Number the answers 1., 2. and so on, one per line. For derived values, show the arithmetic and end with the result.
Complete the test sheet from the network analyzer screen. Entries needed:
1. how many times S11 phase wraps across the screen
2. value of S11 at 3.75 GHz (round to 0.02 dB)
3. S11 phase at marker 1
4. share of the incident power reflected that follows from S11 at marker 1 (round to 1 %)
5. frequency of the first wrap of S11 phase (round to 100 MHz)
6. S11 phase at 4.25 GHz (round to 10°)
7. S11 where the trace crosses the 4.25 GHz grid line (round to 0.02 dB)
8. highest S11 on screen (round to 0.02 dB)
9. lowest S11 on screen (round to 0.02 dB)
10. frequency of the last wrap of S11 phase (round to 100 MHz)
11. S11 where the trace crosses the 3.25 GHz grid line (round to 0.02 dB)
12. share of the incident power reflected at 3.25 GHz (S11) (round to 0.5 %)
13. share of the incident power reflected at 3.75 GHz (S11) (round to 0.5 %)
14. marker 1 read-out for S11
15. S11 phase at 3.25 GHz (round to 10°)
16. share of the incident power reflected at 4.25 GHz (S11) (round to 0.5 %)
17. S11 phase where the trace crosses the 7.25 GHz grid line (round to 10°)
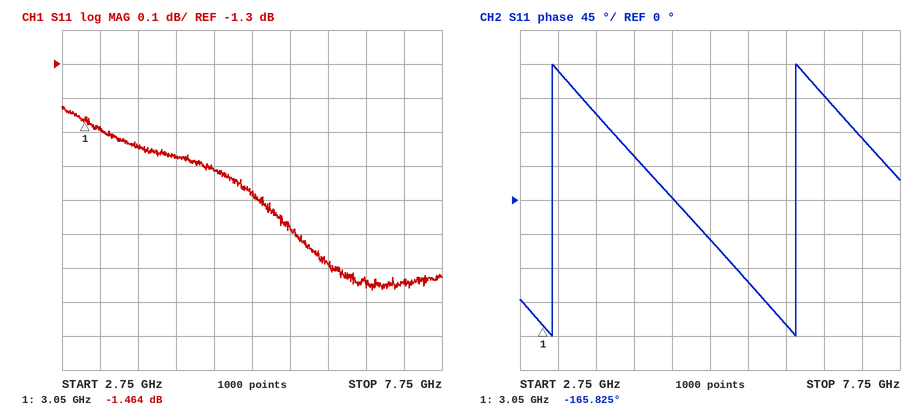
1. 2
2. -1.54 dB
3. -165.825°
4. 10^(-1.464/10) ≈ 71 %
5. 3.2 GHz
6. 60°
7. -1.58 dB
8. -1.42 dB
9. -1.96 dB
10. 6.4 GHz
11. -1.48 dB
12. 10^(-1.48/10) ≈ 71.1 %, so 71.0 % to the nearest 0.5 %
13. 10^(-1.54/10) ≈ 70.1 %, so 70.0 % to the nearest 0.5 %
14. -1.464 dB
15. 170°
16. 10^(-1.58/10) ≈ 69.5 %
17. 80°
